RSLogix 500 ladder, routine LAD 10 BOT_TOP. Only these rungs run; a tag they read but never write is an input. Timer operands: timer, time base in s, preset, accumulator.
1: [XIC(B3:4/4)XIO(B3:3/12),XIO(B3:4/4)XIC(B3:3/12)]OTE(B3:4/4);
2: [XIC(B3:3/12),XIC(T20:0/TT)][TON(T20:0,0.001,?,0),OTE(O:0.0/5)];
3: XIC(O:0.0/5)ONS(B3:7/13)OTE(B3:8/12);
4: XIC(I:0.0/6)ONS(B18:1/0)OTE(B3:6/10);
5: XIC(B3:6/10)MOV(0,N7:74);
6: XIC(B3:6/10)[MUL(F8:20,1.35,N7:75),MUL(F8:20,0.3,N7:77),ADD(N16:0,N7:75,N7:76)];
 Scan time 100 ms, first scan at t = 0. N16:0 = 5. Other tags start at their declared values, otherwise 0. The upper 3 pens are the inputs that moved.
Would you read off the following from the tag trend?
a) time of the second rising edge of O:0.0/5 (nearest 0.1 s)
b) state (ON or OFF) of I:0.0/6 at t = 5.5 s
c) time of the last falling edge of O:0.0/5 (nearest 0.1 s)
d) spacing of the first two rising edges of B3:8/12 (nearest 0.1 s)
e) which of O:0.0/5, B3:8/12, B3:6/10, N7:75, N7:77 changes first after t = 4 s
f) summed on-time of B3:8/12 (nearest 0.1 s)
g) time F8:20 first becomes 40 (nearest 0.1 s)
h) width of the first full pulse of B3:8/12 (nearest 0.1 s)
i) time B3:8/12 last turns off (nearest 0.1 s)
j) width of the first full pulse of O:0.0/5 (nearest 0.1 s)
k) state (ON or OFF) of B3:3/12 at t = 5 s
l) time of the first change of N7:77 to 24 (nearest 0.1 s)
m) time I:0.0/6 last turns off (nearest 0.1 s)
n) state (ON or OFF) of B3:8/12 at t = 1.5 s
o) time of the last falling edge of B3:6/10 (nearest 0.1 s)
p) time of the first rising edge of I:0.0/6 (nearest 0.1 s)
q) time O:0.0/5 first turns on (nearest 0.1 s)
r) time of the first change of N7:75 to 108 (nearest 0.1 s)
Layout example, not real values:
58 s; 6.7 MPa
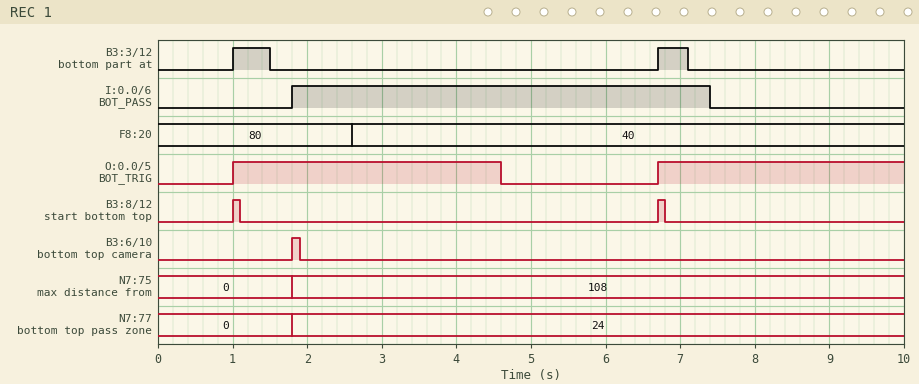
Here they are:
6.7 s; ON; 4.6 s; 5.7 s; O:0.0/5; 0.2 s; 2.6 s; 0.1 s; 6.8 s; 3.6 s; OFF; 1.8 s; 7.4 s; OFF; 1.9 s; 1.8 s; 1.0 s; 1.8 s
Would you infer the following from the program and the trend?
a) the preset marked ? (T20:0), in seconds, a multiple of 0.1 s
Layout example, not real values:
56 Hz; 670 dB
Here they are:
3.5 s
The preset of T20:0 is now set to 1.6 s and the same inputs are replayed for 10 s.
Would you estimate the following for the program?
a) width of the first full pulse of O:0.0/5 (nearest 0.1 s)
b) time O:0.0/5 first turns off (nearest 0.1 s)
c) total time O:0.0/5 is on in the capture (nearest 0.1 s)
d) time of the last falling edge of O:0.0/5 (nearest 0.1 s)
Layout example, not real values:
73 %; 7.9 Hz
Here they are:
1.7 s; 2.7 s; 3.4 s; 8.4 s
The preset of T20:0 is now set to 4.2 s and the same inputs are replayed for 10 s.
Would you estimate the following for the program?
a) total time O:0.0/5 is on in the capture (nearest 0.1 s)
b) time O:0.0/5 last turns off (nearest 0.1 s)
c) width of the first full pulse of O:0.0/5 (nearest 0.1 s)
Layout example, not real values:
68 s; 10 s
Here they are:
7.6 s; 5.3 s; 4.3 s
